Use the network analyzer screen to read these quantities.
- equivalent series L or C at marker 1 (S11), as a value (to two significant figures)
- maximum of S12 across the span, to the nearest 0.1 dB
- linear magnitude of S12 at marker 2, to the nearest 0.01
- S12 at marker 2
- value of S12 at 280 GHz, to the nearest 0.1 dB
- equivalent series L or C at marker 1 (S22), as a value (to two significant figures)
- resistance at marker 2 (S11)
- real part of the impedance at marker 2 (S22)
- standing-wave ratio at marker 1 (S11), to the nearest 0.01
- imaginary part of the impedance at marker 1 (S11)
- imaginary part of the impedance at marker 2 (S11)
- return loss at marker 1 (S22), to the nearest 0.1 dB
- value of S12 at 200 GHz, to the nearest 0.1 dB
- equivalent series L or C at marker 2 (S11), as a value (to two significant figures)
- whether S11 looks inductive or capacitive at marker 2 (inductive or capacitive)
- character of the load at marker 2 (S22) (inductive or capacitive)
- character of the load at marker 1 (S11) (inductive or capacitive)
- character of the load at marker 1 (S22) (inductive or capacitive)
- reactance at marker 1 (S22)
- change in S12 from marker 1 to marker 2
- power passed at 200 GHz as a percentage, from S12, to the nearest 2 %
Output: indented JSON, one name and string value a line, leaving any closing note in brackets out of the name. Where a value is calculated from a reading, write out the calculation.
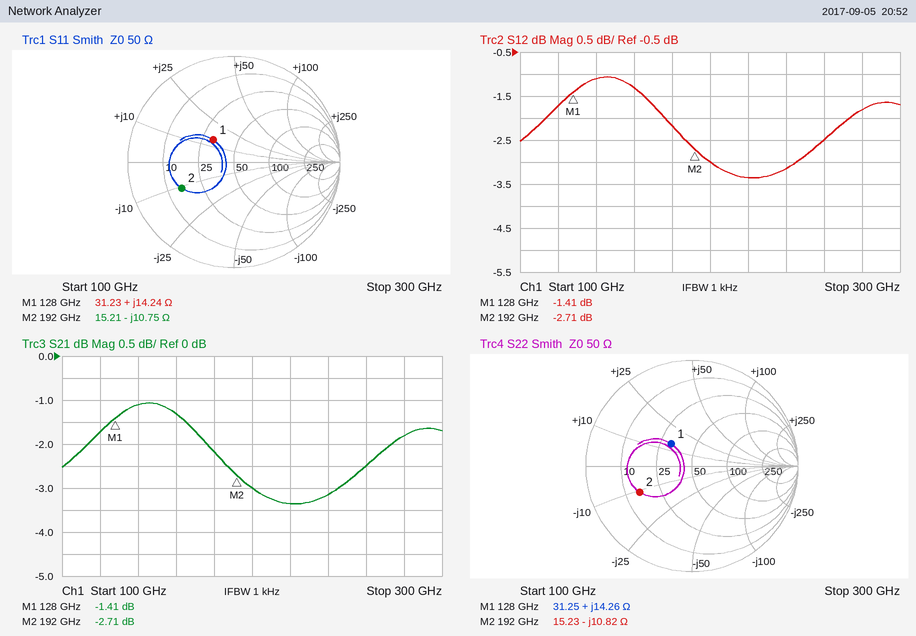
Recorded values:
{
  "equivalent series L or C at marker 1 (S11), as a value": "L = 14.24 Ω/(2π × 128 GHz) ≈ 18 pH",
  "maximum of S12 across the span, to the nearest 0.1 dB": "-1.1 dB",
  "linear magnitude of S12 at marker 2, to the nearest 0.01": "10^(-2.71/20) ≈ 0.73",
  "S12 at marker 2": "-2.71 dB",
  "value of S12 at 280 GHz, to the nearest 0.1 dB": "-1.8 dB",
  "equivalent series L or C at marker 1 (S22), as a value": "L = 14.26 Ω/(2π × 128 GHz) ≈ 18 pH",
  "resistance at marker 2": "15.21 Ω",
  "real part of the impedance at marker 2": "15.23 Ω",
  "standing-wave ratio at marker 1 (S11), to the nearest 0.01": "1.80",
  "imaginary part of the impedance at marker 1": "+14.24 Ω",
  "imaginary part of the impedance at marker 2": "-10.75 Ω",
  "return loss at marker 1 (S22), to the nearest 0.1 dB": "10.9 dB",
  "value of S12 at 200 GHz, to the nearest 0.1 dB": "-3.0 dB",
  "equivalent series L or C at marker 2 (S11), as a value": "C = 1/(2π × 192 GHz × 10.75 Ω) ≈ 77 fF",
  "whether S11 looks inductive or capacitive at marker 2": "capacitive",
  "character of the load at marker 2 (S22)": "capacitive",
  "character of the load at marker 1 (S11)": "inductive",
  "character of the load at marker 1 (S22)": "inductive",
  "reactance at marker 1": "+14.26 Ω",
  "change in S12 from marker 1 to marker 2": "-2.71 − (-1.41) = -1.30 dB",
  "power passed at 200 GHz as a percentage, from S12, to the nearest 2 %": "10^(-3/10) ≈ 50 %"
}
